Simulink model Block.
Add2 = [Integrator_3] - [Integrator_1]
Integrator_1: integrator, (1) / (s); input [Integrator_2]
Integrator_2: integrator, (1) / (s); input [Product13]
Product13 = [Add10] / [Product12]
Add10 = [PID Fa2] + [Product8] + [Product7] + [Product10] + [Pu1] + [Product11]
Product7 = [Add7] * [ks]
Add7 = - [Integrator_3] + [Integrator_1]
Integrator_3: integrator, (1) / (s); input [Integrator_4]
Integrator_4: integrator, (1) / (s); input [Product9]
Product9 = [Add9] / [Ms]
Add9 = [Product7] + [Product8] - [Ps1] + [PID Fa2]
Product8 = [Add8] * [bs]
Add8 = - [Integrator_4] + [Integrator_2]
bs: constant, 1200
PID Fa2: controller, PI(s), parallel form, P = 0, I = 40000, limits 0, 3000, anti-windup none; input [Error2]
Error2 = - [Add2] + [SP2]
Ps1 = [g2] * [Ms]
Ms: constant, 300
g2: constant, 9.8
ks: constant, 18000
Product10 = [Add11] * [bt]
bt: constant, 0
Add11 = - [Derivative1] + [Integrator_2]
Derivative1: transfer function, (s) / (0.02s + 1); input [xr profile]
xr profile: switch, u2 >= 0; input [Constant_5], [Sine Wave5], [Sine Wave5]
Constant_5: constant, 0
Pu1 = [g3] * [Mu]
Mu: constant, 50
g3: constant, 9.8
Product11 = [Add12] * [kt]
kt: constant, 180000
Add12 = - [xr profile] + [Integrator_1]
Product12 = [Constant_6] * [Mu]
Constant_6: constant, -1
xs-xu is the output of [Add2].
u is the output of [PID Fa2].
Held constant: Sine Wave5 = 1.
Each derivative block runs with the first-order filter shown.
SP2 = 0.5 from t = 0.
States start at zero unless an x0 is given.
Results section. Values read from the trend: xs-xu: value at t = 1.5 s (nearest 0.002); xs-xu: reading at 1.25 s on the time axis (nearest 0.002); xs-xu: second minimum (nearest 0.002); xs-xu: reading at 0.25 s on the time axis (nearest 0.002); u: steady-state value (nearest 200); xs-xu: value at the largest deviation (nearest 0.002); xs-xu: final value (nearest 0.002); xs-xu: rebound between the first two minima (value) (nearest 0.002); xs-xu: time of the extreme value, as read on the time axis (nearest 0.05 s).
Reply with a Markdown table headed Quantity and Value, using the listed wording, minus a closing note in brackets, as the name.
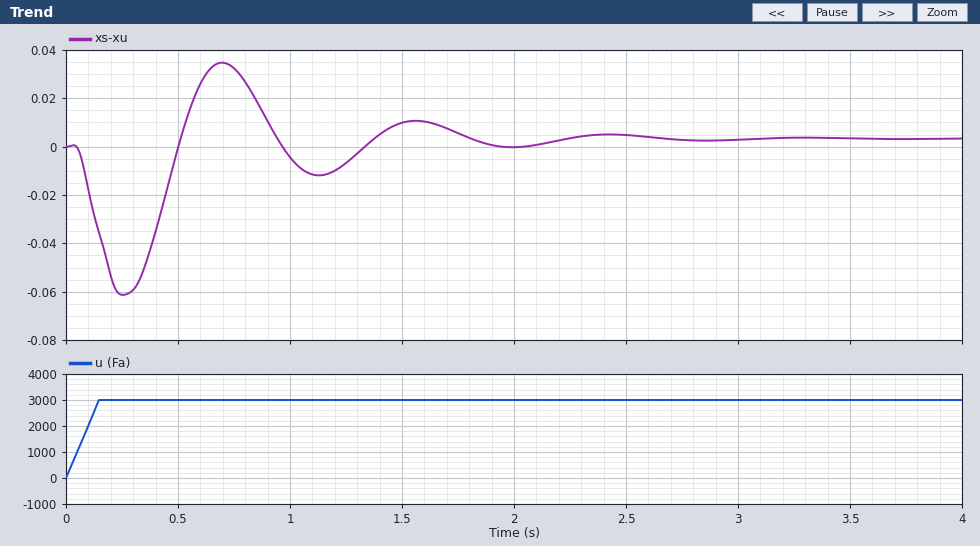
| Quantity | Value |
|---|---|
| xs-xu: value at t = 1.5 s | 0.010 |
| xs-xu: reading at 1.25 s on the time axis | -0.006 |
| xs-xu: second minimum | -0.012 |
| xs-xu: reading at 0.25 s on the time axis | -0.062 |
| u: steady-state value | 3000 |
| xs-xu: value at the largest deviation | -0.062 |
| xs-xu: final value | 0.004 |
| xs-xu: rebound between the first two minima (value) | 0.034 |
| xs-xu: time of the extreme value, as read on the time axis | 0.25 s |
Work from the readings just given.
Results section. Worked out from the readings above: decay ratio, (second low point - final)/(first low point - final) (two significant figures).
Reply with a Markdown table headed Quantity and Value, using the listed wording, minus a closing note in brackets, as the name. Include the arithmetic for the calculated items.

| Quantity | Value |
|---|---|
| decay ratio, (second low point - final)/(first low point - final) | (-0.012 - 0.004) / (-0.062 - 0.004) = 0.24 |
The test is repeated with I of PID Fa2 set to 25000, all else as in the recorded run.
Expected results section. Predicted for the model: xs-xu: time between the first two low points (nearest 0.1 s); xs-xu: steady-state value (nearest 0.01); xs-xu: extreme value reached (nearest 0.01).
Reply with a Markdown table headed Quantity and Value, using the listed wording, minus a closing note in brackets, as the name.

| Quantity | Value |
|---|---|
| xs-xu: time between the first two low points | 0.9 s |
| xs-xu: steady-state value | 0.00 |
| xs-xu: extreme value reached | -0.09 |
